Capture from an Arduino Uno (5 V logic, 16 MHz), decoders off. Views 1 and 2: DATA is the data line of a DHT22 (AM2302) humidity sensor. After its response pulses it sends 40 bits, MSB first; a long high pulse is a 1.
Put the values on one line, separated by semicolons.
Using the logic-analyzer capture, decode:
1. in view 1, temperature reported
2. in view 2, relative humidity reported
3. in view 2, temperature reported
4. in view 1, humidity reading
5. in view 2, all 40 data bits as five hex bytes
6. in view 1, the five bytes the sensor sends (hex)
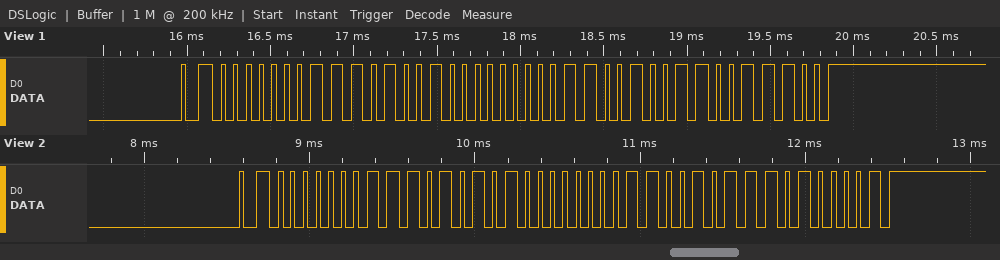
20.1 °C; 46.9 %; 20.3 °C; 46.6 %; 01 D5 00 CB A1; 01 D2 00 C9 9C
